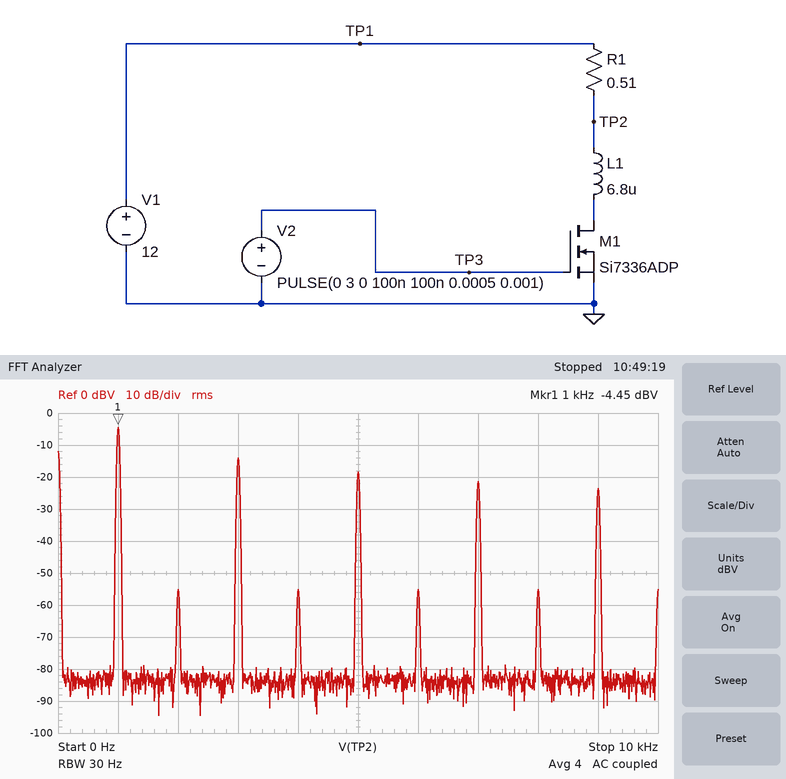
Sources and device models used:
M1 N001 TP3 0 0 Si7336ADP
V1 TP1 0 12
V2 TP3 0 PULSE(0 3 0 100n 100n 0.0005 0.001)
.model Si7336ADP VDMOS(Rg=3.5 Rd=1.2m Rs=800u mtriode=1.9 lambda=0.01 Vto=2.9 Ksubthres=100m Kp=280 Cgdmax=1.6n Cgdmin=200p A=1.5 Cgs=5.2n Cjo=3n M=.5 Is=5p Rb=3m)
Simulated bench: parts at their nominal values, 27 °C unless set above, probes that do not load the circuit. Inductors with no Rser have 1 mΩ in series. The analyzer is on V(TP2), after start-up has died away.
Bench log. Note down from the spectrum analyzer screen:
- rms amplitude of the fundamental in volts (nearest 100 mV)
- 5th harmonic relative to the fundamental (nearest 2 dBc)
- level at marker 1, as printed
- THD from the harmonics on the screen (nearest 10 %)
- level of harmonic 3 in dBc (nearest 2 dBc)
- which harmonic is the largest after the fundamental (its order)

600 mV
-14 dBc
-4.45 dBV
40 %
-10 dBc
3
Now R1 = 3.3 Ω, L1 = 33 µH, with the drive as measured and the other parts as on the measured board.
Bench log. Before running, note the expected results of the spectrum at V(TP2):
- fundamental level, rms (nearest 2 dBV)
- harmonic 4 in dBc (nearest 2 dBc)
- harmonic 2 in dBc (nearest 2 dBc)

12 dBV
-34 dBc
-34 dBc
